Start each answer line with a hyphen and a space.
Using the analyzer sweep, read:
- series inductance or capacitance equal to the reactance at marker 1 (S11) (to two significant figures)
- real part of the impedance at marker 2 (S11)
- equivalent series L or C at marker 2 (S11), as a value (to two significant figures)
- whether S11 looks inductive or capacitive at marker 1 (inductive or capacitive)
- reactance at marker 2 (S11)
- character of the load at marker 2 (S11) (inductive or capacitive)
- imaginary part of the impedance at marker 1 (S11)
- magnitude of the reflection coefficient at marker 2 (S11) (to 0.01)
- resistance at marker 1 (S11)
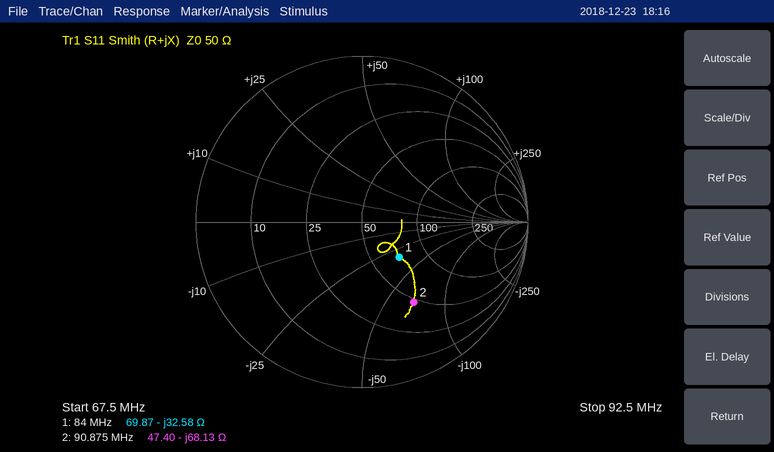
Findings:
- 58 pF
- 47.40 Ω
- 26 pF
- capacitive
- -68.13 Ω
- capacitive
- -32.58 Ω
- 0.57
- 69.87 Ω
